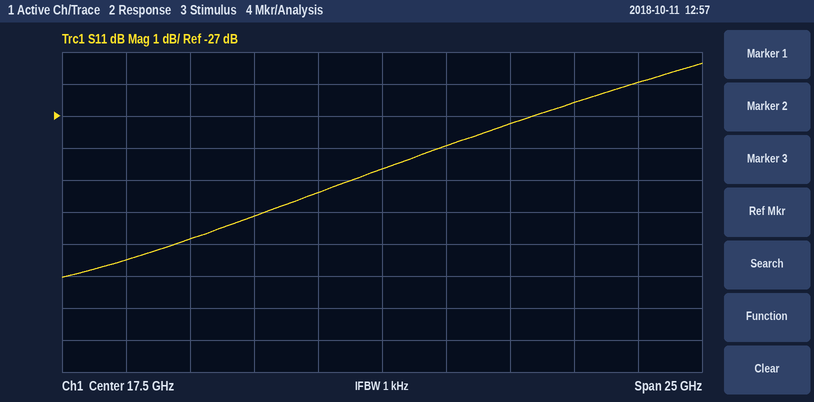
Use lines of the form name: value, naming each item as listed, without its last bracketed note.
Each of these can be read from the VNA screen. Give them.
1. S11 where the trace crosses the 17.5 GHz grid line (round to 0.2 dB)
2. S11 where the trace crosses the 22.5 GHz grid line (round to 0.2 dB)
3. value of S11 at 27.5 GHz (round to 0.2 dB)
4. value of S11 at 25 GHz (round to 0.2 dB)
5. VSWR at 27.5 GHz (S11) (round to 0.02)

S11 where the trace crosses the 17.5 GHz grid line: -28.6 dB
S11 where the trace crosses the 22.5 GHz grid line: -27.2 dB
value of S11 at 27.5 GHz: -26.0 dB
value of S11 at 25 GHz: -26.6 dB
VSWR at 27.5 GHz (S11): 1.10
